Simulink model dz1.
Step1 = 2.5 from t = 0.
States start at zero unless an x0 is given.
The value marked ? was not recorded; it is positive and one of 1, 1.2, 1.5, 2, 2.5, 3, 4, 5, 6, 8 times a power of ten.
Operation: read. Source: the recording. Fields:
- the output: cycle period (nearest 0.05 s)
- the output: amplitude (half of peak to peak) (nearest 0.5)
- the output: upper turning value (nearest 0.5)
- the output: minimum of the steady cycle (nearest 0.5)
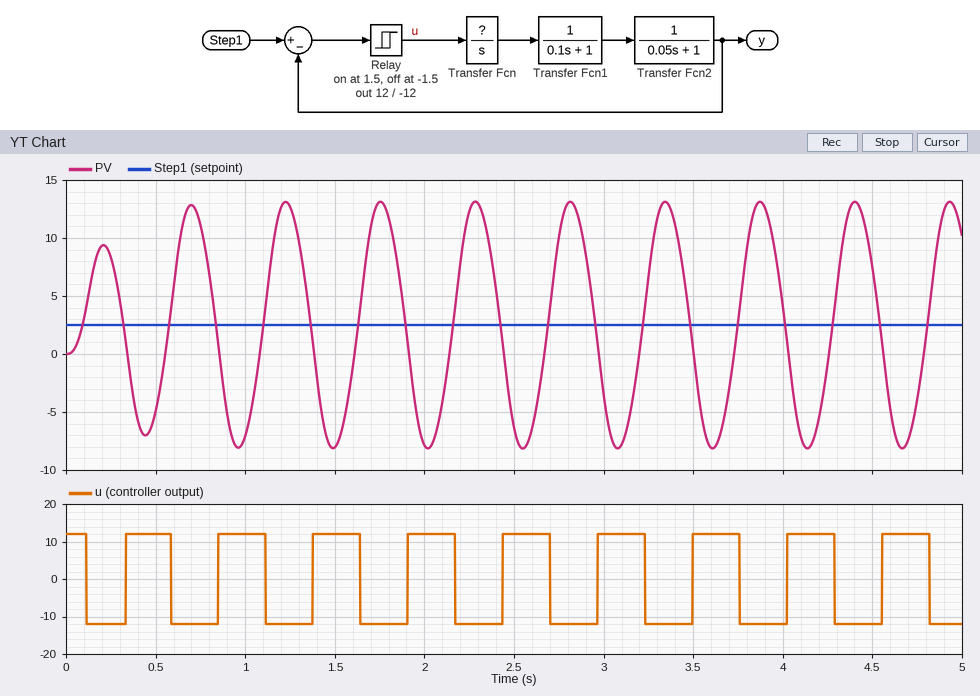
0.55 s
10.5
13.0
-8.0
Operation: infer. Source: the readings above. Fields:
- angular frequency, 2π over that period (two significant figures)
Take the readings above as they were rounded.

11 rad/s
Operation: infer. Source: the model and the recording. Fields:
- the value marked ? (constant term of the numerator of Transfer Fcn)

15
